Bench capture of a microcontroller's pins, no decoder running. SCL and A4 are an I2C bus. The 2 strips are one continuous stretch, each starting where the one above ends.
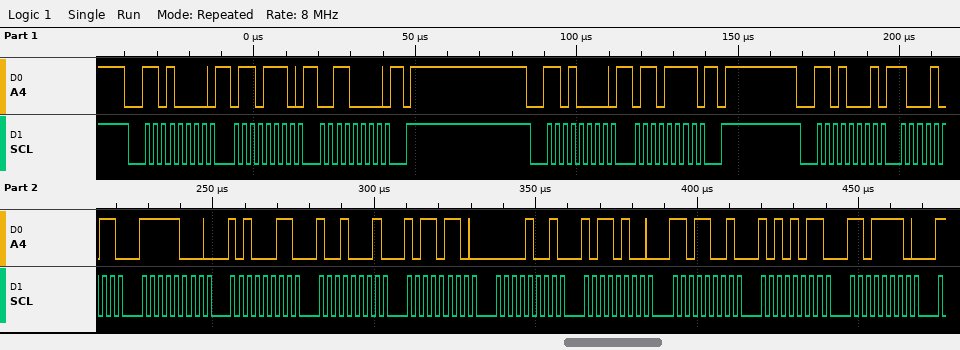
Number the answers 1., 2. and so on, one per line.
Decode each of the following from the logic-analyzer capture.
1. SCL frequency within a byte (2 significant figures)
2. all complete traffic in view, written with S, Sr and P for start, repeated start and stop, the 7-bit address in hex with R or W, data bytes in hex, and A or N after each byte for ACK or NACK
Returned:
1. 400 kHz
2. S 68W A 6E A 30 A P S 68W A 6F A P S 68R A 8B A F8 A A3 A 91 A B6 A 09 A B4 A D9 A AB A DE A
